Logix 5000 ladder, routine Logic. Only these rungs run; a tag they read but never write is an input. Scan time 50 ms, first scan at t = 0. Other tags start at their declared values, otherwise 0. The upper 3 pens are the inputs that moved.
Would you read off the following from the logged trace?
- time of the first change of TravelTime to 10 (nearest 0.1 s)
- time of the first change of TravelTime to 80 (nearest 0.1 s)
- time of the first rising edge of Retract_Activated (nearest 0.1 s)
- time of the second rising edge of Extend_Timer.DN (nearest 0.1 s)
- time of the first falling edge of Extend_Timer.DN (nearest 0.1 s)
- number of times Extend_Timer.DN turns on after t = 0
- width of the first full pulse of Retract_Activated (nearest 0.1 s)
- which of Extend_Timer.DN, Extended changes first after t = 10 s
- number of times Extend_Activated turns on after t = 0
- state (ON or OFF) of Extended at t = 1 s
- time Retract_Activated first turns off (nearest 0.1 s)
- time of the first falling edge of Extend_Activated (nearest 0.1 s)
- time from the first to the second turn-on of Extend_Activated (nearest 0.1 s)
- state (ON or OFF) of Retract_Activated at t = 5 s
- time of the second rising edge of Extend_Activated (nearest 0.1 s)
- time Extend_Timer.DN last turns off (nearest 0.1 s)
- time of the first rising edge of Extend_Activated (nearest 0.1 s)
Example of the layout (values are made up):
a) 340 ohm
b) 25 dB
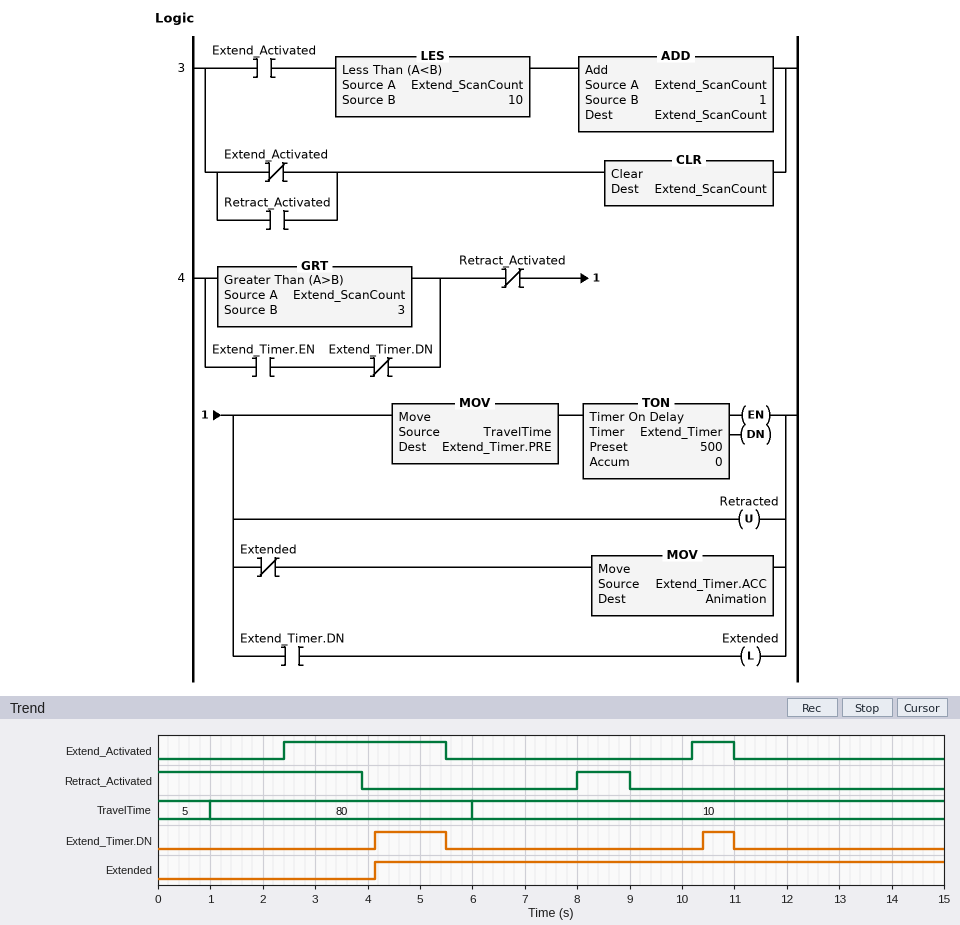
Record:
a) 6.0 s
b) 1.0 s
c) 8.0 s
d) 10.4 s
e) 5.5 s
f) 2
g) 1.0 s
h) Extend_Timer.DN
i) 2
j) OFF
k) 3.9 s
l) 5.5 s
m) 7.8 s
n) OFF
o) 10.2 s
p) 11.0 s
q) 2.4 s
